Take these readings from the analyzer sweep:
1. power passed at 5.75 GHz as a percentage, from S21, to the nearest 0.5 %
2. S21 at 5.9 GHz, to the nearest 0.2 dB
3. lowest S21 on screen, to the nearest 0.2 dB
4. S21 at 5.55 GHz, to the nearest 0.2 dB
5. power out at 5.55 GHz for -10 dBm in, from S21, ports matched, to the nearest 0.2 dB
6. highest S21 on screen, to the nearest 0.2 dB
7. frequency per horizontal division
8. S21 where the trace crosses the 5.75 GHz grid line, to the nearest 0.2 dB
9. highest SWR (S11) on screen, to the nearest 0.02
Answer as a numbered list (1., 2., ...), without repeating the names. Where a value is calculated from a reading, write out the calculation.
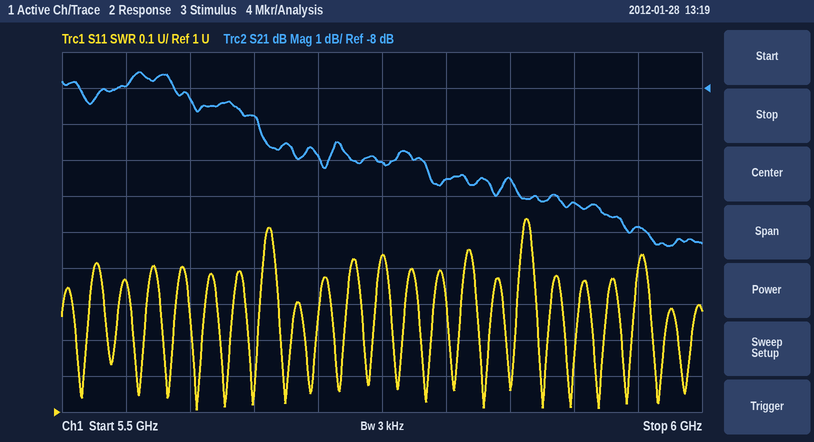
1. 10^(-10/10) ≈ 10.0 %
2. -11.2 dB
3. -12.4 dB
4. -8.0 dB
5. -10 dBm + (-8.0 dB) = -18.0 dBm
6. -7.6 dB
7. 50 MHz
8. -10.0 dB
9. 1.54
